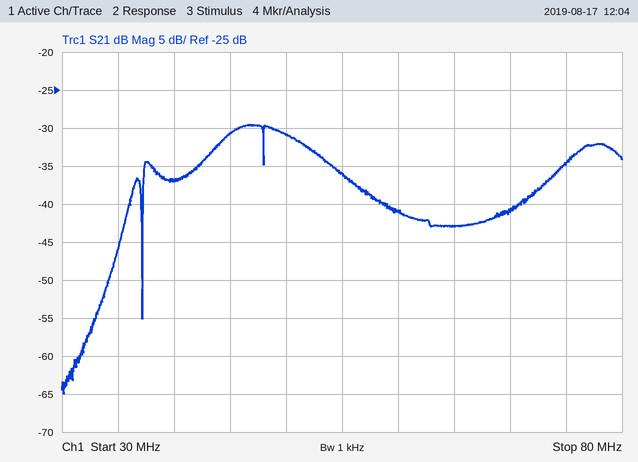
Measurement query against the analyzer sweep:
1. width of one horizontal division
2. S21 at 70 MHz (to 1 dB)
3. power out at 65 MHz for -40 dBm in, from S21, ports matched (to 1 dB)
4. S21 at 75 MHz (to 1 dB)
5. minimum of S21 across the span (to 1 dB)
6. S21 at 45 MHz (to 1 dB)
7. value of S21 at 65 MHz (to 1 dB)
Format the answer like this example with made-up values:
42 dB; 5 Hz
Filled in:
5 MHz; -41 dB; -83 dBm; -35 dB; -65 dB; -31 dB; -43 dB
